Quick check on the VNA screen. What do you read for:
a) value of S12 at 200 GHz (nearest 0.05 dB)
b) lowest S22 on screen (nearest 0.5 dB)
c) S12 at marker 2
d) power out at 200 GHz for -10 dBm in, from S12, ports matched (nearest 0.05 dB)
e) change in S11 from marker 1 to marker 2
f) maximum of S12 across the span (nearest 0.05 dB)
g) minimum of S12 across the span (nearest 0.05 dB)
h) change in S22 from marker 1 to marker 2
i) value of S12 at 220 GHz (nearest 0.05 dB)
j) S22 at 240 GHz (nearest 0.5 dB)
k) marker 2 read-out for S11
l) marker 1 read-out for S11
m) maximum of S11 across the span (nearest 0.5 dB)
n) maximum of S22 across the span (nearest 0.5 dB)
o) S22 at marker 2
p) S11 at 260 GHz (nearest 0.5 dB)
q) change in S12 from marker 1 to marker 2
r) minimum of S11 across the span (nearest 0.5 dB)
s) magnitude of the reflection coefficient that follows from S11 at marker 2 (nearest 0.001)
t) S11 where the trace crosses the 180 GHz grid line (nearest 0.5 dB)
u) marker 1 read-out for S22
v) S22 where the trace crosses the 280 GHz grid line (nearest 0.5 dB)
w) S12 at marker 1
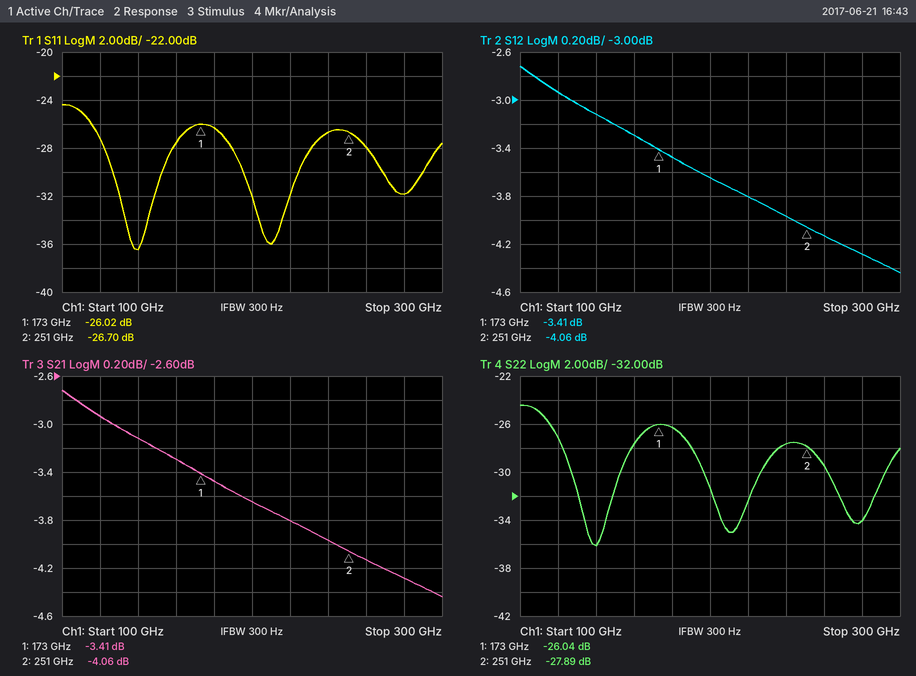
-3.65 dB
-36.0 dB
-4.06 dB
-13.65 dBm
-0.68 dB
-2.70 dB
-4.45 dB
-1.85 dB
-3.80 dB
-27.5 dB
-26.70 dB
-26.02 dB
-24.5 dB
-24.5 dB
-27.89 dB
-28.0 dB
-0.65 dB
-36.5 dB
0.046
-26.5 dB
-26.04 dB
-34.0 dB
-3.41 dB
